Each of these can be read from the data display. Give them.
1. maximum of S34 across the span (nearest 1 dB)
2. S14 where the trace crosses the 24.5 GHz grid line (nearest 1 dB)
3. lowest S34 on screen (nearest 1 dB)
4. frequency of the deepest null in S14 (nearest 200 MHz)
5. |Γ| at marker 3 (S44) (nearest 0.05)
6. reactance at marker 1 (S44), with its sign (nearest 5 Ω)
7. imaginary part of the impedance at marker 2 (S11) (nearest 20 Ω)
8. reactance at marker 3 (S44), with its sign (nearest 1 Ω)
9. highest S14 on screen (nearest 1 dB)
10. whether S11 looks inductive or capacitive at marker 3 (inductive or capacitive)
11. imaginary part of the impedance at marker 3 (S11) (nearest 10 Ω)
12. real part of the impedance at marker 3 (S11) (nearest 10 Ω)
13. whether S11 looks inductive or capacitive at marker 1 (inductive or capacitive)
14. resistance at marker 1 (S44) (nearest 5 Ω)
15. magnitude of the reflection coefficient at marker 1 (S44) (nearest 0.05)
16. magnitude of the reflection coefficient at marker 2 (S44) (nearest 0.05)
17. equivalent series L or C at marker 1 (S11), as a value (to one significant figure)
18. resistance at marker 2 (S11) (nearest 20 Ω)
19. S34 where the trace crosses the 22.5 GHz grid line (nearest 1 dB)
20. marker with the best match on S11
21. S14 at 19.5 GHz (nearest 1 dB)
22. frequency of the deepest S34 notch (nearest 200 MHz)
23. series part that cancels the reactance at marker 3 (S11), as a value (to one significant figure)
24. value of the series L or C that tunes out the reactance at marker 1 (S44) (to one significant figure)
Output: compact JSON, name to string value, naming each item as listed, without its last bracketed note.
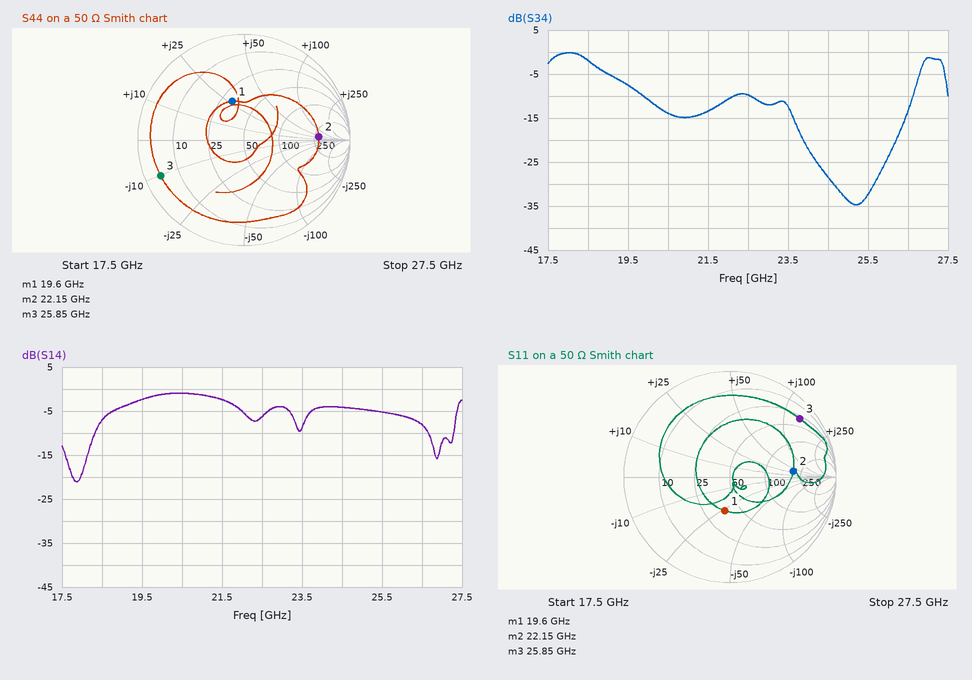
{"maximum of S34 across the span": "0 dB", "S14 where the trace crosses the 24.5 GHz grid line": "-4 dB", "lowest S34 on screen": "-35 dB", "frequency of the deepest null in S14": "17.8 GHz", "|Γ| at marker 3 (S44)": "0.85", "reactance at marker 1 (S44), with its sign": "+25 Ω", "imaginary part of the impedance at marker 2 (S11)": "+40 Ω", "reactance at marker 3 (S44), with its sign": "-10 Ω", "highest S14 on screen": "-1 dB", "whether S11 looks inductive or capacitive at marker 3": "inductive", "imaginary part of the impedance at marker 3 (S11)": "+130 Ω", "real part of the impedance at marker 3 (S11)": "30 Ω", "whether S11 looks inductive or capacitive at marker 1": "capacitive", "resistance at marker 1 (S44)": "30 Ω", "magnitude of the reflection coefficient at marker 1 (S44)": "0.40", "magnitude of the reflection coefficient at marker 2 (S44)": "0.70", "equivalent series L or C at marker 1 (S11), as a value": "300 fF", "resistance at marker 2 (S11)": "200 Ω", "S34 where the trace crosses the 22.5 GHz grid line": "-10 dB", "marker with the best match on S11": "marker 1", "S14 at 19.5 GHz": "-2 dB", "frequency of the deepest S34 notch": "25.2 GHz", "series part that cancels the reactance at marker 3 (S11), as a value": "50 fF", "value of the series L or C that tunes out the reactance at marker 1 (S44)": "300 fF"}
